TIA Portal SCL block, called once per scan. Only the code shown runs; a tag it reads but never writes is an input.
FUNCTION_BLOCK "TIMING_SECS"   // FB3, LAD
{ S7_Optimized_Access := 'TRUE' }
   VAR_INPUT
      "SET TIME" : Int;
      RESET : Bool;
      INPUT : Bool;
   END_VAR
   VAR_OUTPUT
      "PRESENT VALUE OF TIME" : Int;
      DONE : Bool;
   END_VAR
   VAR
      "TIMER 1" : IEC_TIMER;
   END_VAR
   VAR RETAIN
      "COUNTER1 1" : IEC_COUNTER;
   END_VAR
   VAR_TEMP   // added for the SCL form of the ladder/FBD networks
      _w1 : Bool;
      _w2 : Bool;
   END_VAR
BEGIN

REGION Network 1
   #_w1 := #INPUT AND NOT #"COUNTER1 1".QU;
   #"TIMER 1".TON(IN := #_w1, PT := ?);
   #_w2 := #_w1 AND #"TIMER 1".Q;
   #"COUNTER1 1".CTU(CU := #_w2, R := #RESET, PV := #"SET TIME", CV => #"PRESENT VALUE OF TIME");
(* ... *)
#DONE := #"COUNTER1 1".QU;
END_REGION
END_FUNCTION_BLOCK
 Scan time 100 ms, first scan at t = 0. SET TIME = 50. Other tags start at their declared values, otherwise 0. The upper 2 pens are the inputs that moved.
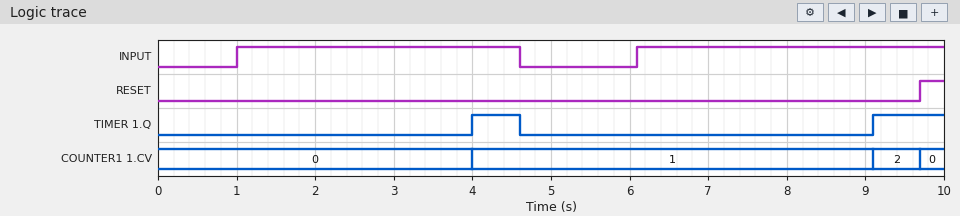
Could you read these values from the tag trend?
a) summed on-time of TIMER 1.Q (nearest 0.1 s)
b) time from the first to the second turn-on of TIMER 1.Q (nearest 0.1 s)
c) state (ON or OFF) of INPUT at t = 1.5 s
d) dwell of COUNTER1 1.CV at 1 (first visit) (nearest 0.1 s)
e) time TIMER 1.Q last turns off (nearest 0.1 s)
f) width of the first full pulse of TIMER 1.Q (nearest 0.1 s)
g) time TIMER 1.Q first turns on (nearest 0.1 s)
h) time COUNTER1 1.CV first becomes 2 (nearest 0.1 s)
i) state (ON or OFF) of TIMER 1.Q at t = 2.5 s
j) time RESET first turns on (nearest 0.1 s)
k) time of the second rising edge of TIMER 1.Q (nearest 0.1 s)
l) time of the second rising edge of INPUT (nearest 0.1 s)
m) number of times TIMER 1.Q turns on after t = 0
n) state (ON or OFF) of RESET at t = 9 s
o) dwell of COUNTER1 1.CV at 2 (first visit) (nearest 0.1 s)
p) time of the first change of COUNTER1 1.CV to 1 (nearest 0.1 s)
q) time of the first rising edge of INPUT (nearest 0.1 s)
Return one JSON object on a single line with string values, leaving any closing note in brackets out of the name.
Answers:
{"summed on-time of TIMER 1.Q": "1.5 s", "time from the first to the second turn-on of TIMER 1.Q": "5.1 s", "state (ON or OFF) of INPUT at t = 1.5 s": "ON", "dwell of COUNTER1 1.CV at 1 (first visit)": "5.1 s", "time TIMER 1.Q last turns off": "4.6 s", "width of the first full pulse of TIMER 1.Q": "0.6 s", "time TIMER 1.Q first turns on": "4.0 s", "time COUNTER1 1.CV first becomes 2": "9.1 s", "state (ON or OFF) of TIMER 1.Q at t = 2.5 s": "OFF", "time RESET first turns on": "9.7 s", "time of the second rising edge of TIMER 1.Q": "9.1 s", "time of the second rising edge of INPUT": "6.1 s", "number of times TIMER 1.Q turns on after t = 0": "2", "state (ON or OFF) of RESET at t = 9 s": "OFF", "dwell of COUNTER1 1.CV at 2 (first visit)": "0.6 s", "time of the first change of COUNTER1 1.CV to 1": "4.0 s", "time of the first rising edge of INPUT": "1.0 s"}
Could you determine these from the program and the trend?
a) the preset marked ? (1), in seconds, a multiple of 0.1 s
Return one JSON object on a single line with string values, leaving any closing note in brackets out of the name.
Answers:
{"the preset marked ? (1), in seconds, a multiple of 0.1 s": "3.0 s"}
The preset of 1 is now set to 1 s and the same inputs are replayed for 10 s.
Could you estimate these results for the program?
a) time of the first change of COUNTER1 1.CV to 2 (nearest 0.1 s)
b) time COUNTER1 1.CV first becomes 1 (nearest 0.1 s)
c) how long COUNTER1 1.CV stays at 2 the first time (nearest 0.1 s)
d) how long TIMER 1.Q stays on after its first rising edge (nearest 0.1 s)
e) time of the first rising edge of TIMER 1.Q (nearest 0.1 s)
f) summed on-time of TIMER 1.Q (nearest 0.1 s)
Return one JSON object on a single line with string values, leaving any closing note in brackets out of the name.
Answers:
{"time of the first change of COUNTER1 1.CV to 2": "7.1 s", "time COUNTER1 1.CV first becomes 1": "2.0 s", "how long COUNTER1 1.CV stays at 2 the first time": "2.6 s", "how long TIMER 1.Q stays on after its first rising edge": "2.6 s", "time of the first rising edge of TIMER 1.Q": "2.0 s", "summed on-time of TIMER 1.Q": "5.5 s"}
